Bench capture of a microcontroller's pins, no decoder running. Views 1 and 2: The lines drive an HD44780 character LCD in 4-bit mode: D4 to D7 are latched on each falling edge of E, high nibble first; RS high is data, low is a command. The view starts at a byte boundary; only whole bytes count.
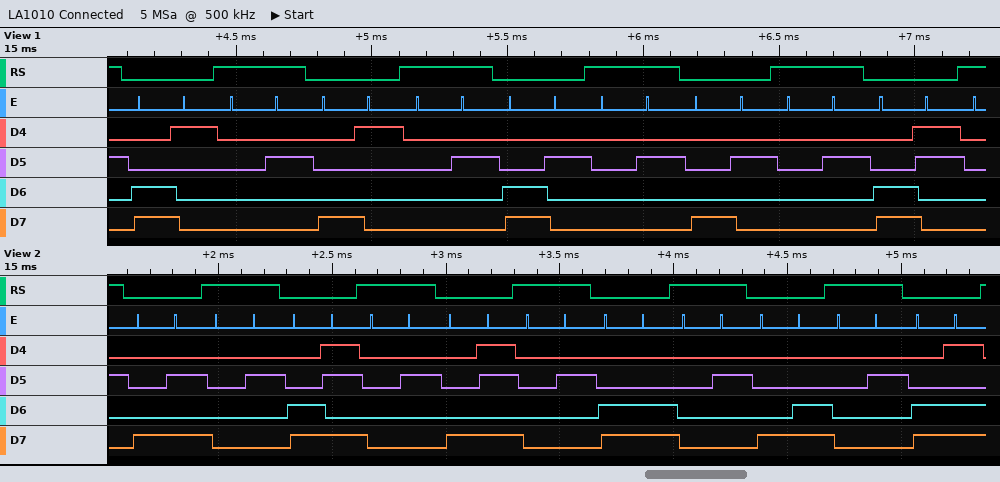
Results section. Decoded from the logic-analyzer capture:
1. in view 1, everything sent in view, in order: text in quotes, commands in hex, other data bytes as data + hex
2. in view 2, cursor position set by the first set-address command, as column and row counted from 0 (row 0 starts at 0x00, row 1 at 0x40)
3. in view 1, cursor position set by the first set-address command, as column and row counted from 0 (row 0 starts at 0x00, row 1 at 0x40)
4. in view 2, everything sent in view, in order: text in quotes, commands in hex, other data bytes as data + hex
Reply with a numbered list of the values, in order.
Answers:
1. 0xC1 data 02 0x81 data 02 0xC2 data 02 0x82 data 02 0xC3
2. column 10, row 0
3. column 1, row 1
4. 0x8A data 02 0xCB data 02 0x8B data 02 0xCC data 02 0x8C data 02 0xCD
